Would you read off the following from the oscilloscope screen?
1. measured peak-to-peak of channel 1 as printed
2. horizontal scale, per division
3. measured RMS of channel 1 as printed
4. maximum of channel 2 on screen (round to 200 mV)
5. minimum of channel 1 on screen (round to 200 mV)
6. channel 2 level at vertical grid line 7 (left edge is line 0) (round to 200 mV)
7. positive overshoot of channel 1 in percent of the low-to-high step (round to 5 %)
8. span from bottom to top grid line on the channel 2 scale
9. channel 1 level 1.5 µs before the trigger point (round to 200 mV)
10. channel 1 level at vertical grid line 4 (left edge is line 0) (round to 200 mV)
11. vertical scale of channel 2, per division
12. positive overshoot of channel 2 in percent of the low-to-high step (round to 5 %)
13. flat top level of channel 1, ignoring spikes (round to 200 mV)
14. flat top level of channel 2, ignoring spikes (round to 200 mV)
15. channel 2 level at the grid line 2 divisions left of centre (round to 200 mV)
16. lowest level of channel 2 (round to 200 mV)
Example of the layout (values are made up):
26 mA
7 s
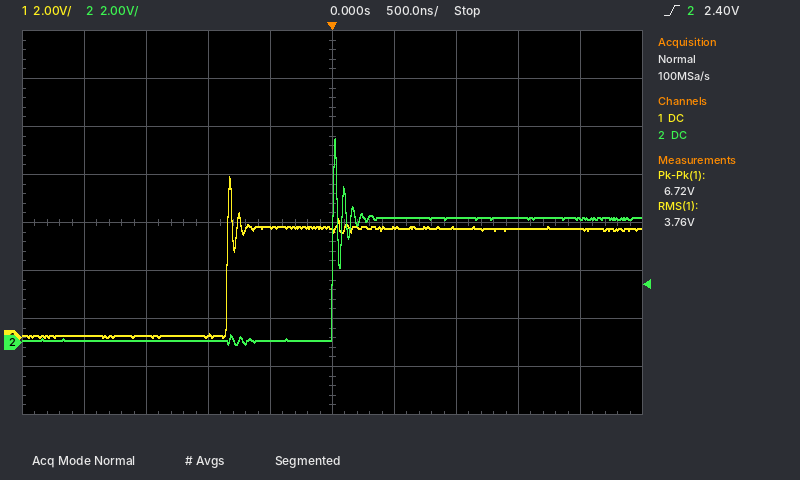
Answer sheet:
6.72 V
500 ns
3.76 V
8.4 V
0.0 V
5.2 V
50 %
16 V
0.0 V
4.6 V
2 V
65 %
4.6 V
5.2 V
0.0 V
0.0 V
